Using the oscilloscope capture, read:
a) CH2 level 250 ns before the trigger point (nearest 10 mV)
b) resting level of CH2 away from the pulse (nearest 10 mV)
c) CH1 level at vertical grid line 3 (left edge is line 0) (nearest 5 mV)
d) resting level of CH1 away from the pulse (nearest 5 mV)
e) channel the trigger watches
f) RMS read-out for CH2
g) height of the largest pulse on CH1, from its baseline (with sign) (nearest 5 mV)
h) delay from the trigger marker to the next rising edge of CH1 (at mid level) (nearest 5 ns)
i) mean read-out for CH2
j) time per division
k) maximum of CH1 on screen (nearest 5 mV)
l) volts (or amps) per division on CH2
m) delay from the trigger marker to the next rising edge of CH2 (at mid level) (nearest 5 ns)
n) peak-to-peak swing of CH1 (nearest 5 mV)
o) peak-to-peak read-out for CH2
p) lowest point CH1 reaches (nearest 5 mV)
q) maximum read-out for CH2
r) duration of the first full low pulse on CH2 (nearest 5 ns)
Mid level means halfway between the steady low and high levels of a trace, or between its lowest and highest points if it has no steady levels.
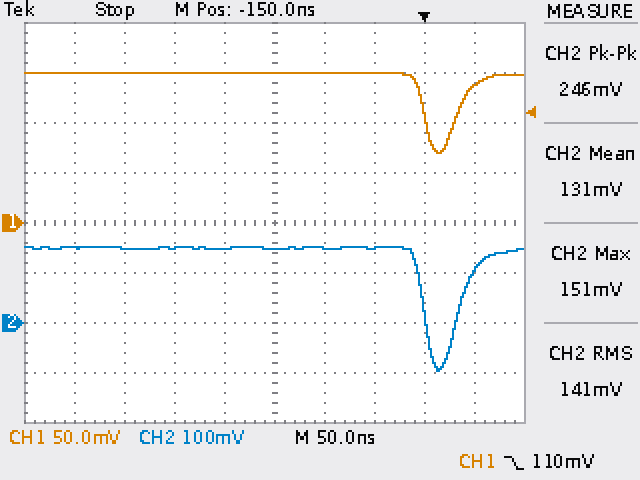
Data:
150 mV
150 mV
150 mV
150 mV
CH1
141 mV
-80 mV
35 ns
131 mV
50 ns
150 mV
100 mV
35 ns
80 mV
246 mV
70 mV
151 mV
35 ns
